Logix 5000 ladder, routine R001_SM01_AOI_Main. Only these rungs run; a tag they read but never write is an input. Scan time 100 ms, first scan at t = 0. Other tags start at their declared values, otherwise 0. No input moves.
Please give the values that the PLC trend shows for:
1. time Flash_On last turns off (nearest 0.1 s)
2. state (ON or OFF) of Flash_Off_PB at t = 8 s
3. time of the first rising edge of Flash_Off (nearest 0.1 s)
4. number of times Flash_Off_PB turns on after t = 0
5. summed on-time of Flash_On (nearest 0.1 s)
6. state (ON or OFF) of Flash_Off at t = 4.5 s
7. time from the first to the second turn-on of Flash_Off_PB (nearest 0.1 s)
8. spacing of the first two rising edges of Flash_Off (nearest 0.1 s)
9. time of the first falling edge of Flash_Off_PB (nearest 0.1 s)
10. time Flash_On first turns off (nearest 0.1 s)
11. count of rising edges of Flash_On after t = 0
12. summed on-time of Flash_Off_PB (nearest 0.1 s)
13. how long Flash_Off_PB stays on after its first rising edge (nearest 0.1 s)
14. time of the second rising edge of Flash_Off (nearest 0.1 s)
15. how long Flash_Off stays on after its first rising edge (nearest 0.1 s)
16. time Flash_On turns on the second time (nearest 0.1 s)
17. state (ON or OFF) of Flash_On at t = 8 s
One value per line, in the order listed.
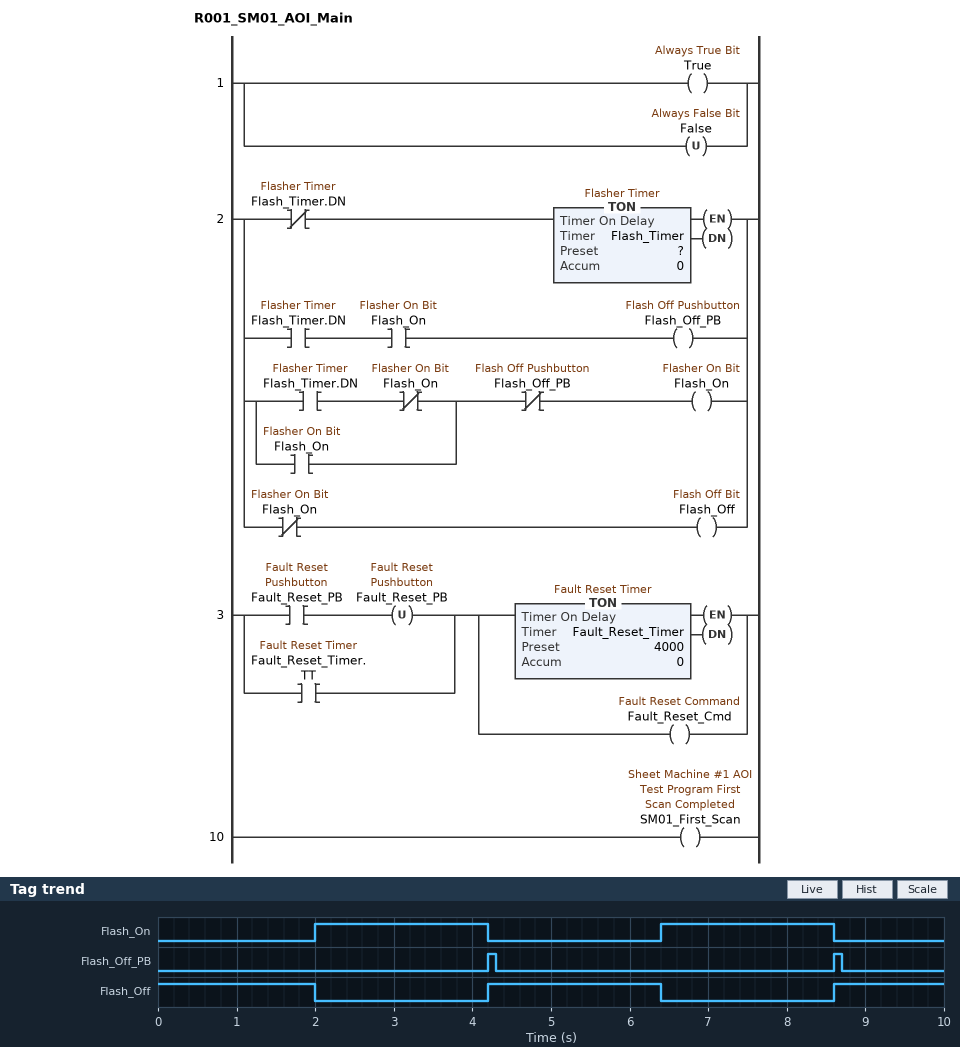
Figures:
8.6 s
OFF
4.2 s
2
4.4 s
ON
4.4 s
4.4 s
4.3 s
4.2 s
2
0.2 s
0.1 s
8.6 s
2.2 s
6.4 s
ON
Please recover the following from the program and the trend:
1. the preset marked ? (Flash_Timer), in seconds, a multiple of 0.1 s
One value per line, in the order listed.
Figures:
2.0 s
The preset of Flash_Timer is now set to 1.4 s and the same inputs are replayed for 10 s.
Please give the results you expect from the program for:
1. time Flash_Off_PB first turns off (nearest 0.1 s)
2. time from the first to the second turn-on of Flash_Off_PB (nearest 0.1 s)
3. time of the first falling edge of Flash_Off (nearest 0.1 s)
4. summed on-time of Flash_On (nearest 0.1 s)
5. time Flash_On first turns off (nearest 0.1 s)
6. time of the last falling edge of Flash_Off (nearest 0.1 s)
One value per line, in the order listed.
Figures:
3.1 s
3.2 s
1.4 s
4.8 s
3.0 s
7.8 s
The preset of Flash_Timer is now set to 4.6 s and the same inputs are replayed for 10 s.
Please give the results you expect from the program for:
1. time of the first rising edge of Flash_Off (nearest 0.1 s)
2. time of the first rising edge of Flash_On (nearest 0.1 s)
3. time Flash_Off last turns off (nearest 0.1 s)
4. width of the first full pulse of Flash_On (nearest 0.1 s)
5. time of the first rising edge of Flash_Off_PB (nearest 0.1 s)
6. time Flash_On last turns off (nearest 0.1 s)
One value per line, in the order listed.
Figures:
9.4 s
4.6 s
4.6 s
4.8 s
9.4 s
9.4 s
